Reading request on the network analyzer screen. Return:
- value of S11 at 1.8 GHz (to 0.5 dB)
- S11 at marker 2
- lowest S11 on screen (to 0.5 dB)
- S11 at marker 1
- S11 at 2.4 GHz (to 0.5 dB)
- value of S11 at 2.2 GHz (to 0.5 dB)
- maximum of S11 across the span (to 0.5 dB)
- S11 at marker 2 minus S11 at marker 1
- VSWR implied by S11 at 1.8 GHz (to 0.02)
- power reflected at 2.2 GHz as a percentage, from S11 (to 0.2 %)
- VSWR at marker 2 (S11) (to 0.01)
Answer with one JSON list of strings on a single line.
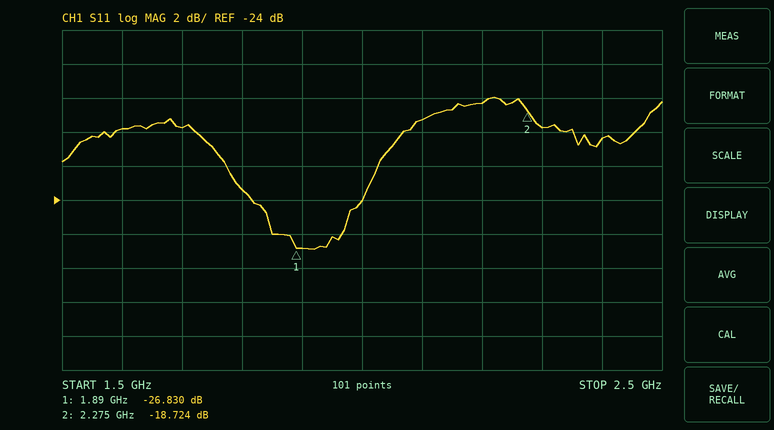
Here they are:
["-23.5 dB", "-18.724 dB", "-27.0 dB", "-26.830 dB", "-20.5 dB", "-18.5 dB", "-18.0 dB", "8.106 dB", "1.14", "1.4 %", "1.26"]
